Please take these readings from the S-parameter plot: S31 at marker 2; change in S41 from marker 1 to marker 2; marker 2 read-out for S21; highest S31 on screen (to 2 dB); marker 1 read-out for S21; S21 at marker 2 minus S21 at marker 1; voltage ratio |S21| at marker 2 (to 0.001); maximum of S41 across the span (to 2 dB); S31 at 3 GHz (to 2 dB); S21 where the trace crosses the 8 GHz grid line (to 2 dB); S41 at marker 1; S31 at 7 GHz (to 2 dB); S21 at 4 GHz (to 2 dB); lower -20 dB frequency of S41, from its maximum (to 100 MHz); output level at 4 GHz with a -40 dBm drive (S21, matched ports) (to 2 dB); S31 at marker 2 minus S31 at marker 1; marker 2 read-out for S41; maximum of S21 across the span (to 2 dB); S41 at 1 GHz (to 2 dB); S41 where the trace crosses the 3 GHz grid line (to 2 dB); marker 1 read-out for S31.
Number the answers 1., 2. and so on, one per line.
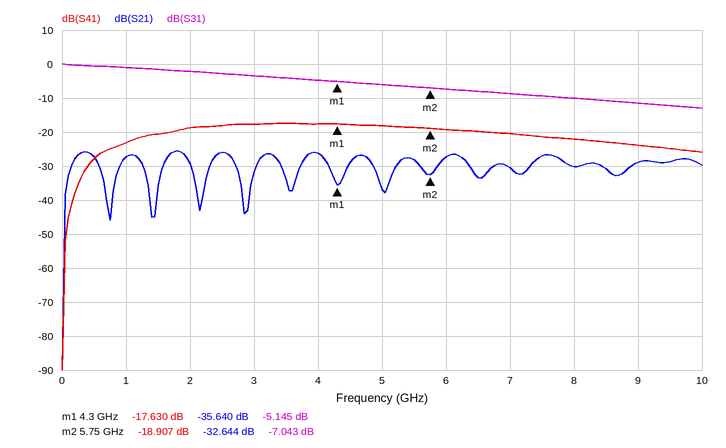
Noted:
1. -7.043 dB
2. -1.277 dB
3. -32.644 dB
4. 0 dB
5. -35.640 dB
6. 2.996 dB
7. 0.023
8. -18 dB
9. -4 dB
10. -30 dB
11. -17.630 dB
12. -8 dB
13. -26 dB
14. 200 MHz
15. -66 dBm
16. -1.898 dB
17. -18.907 dB
18. -26 dB
19. -24 dB
20. -18 dB
21. -5.145 dB
